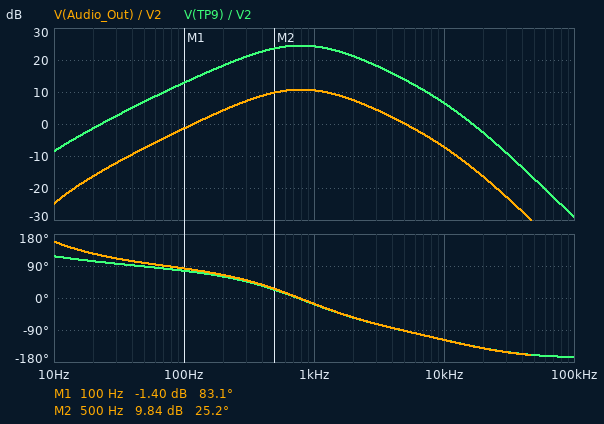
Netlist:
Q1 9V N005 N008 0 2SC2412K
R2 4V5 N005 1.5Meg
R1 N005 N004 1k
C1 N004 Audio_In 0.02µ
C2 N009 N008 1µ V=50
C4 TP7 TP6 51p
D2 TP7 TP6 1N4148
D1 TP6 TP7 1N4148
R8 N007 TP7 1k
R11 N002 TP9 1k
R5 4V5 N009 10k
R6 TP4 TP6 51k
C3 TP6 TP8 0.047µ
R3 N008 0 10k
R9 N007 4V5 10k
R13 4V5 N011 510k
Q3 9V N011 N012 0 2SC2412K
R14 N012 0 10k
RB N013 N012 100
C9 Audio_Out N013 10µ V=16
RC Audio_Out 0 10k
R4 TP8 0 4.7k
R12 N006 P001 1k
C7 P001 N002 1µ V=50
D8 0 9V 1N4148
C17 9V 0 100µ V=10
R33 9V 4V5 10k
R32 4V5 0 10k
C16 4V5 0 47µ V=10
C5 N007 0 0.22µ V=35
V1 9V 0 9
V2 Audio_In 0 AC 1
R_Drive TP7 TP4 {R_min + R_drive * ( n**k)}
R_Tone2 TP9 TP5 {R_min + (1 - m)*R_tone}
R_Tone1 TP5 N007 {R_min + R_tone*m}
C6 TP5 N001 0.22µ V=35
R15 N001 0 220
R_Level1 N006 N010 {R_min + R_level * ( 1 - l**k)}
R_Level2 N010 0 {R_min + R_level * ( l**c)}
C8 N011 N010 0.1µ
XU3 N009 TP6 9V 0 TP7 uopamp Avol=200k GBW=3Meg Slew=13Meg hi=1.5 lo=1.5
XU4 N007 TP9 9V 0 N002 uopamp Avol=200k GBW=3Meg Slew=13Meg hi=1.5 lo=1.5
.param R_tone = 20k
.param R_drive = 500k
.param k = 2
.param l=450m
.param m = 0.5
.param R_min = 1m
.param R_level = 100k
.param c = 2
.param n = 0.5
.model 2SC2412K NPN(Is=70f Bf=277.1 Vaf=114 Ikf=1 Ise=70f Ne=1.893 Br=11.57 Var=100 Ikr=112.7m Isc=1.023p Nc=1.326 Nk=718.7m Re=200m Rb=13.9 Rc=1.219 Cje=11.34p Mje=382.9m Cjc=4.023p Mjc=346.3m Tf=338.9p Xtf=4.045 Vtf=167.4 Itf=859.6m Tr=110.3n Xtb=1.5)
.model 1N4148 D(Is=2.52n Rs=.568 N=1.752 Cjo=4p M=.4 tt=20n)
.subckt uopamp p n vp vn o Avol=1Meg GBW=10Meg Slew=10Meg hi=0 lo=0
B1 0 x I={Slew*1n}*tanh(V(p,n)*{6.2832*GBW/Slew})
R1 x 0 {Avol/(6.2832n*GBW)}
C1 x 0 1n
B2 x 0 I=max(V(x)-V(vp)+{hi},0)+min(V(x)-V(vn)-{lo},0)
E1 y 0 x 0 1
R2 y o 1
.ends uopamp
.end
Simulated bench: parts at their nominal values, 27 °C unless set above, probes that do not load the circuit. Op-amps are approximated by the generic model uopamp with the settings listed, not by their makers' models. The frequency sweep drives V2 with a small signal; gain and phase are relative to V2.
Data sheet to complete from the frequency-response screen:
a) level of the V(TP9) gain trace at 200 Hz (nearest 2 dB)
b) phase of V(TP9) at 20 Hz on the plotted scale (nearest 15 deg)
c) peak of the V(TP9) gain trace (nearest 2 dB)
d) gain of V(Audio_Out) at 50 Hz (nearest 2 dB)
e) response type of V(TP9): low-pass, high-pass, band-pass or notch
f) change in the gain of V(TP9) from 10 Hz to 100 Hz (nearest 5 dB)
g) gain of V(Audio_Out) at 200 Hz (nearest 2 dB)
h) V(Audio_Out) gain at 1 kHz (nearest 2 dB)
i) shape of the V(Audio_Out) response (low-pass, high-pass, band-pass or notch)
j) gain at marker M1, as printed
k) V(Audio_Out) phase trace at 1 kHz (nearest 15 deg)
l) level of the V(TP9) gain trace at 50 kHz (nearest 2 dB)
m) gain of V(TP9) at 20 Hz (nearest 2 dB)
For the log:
18 dB
105 deg
24 dB
-8 dB
band-pass
20 dB
4 dB
10 dB
band-pass
-1.40 dB
-15 deg
-18 dB
-2 dB
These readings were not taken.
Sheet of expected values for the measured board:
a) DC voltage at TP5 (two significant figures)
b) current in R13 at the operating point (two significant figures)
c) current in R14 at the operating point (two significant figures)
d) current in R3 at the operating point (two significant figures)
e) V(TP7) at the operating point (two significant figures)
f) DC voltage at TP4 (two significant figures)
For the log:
4.5 V
1.2 µA
330 µA
260 µA
4.5 V
4.5 V
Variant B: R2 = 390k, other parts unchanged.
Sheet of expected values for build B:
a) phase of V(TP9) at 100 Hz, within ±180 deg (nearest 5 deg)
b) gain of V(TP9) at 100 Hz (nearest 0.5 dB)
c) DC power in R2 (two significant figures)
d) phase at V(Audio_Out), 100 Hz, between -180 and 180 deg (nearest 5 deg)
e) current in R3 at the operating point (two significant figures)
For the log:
85 deg
12.5 dB
560 nW
90 deg
340 µA
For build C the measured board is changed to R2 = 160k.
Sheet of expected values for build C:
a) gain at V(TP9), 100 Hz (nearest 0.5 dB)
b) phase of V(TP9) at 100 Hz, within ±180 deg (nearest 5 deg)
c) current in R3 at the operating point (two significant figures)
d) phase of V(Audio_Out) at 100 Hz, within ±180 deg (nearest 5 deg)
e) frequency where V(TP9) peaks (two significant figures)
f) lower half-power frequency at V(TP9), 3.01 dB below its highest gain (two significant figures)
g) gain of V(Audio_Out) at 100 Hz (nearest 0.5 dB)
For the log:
12.0 dB
100 deg
370 µA
105 deg
800 Hz
330 Hz
-2.5 dB
